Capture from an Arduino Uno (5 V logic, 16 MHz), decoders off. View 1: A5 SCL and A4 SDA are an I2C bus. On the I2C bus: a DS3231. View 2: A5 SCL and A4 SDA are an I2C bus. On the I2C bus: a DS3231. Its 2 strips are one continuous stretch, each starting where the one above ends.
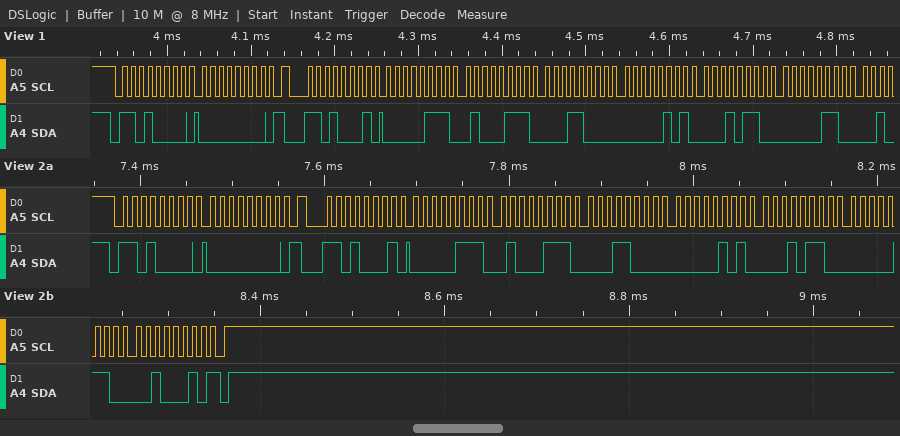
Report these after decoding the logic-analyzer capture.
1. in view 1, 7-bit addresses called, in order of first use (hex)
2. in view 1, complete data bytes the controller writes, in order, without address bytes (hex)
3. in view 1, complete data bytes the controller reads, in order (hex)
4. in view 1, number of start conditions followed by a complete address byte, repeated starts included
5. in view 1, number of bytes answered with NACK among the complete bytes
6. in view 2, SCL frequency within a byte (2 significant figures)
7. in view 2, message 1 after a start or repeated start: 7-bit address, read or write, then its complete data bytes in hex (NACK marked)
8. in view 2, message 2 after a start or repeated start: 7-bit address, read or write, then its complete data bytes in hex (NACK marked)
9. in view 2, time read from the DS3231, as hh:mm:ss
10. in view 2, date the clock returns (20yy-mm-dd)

0x68
00
07 47 18 05 16 06
2
0
100 kHz
0x68 write: 00
0x68 read: 07 47 18 05 16 06 22 NACK
18:47:07
2022-06-16
